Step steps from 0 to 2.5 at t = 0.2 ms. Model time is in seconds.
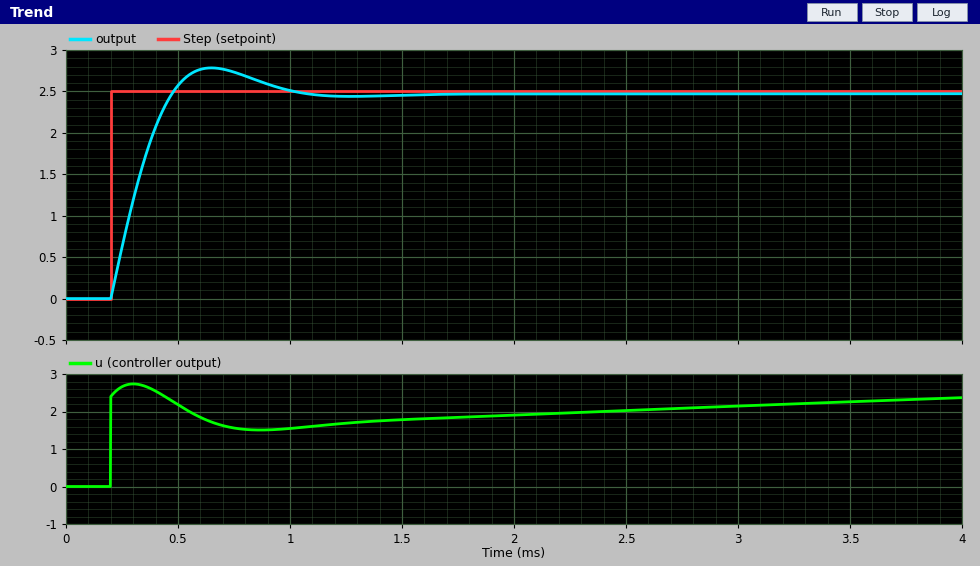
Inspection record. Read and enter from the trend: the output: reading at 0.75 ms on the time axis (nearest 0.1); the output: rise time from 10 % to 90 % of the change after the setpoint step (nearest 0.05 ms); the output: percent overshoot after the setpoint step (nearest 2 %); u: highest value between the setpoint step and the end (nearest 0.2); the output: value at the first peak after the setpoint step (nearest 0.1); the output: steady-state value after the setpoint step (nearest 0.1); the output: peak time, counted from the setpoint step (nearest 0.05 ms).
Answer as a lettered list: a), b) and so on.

a) 2.7
b) 0.20 ms
c) 12 %
d) 2.8
e) 2.8
f) 2.5
g) 0.45 ms
